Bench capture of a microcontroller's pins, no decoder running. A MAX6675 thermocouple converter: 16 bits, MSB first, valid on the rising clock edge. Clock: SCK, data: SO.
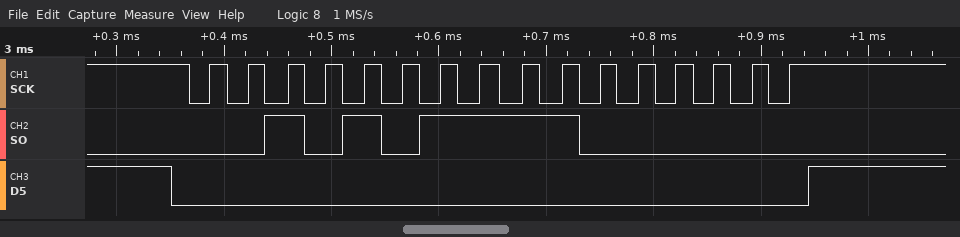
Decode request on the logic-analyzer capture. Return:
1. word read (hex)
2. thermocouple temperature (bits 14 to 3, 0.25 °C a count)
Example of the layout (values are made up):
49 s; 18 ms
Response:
0x2BC0; 350.00 °C
